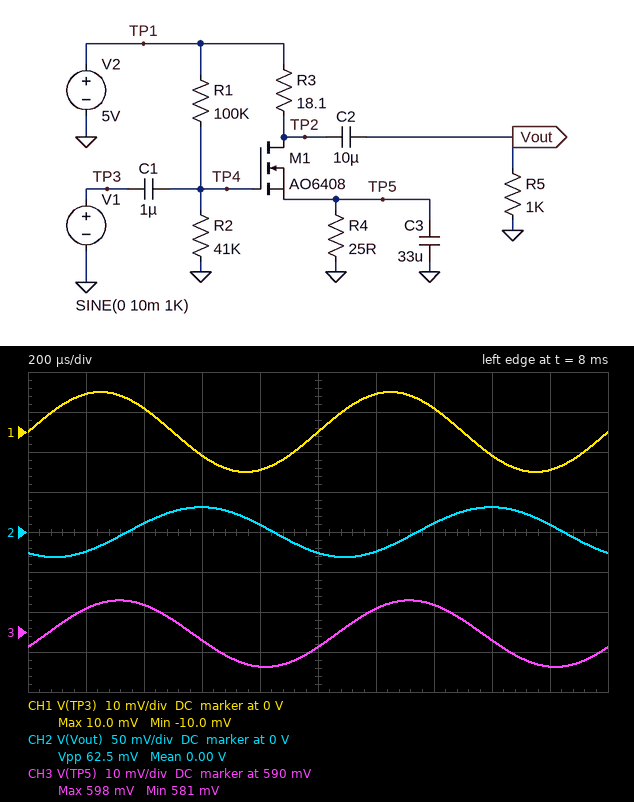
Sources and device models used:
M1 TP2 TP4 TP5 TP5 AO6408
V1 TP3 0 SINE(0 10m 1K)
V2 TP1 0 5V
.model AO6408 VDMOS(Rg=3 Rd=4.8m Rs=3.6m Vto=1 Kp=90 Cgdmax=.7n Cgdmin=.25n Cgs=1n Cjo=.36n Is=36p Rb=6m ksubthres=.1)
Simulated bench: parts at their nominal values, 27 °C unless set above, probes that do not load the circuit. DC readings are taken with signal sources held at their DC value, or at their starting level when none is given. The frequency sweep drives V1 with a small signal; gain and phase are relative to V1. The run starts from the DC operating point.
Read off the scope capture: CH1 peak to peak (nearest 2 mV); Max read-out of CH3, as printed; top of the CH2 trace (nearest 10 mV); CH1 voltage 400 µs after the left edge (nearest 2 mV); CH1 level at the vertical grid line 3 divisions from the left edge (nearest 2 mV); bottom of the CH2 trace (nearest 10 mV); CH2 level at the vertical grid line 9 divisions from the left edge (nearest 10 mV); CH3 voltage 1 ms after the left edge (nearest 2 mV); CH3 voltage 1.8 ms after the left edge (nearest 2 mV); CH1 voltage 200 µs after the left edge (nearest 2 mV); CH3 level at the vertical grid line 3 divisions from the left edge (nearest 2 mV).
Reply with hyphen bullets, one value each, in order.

- 20 mV
- 598 mV
- 30 mV
- 6 mV
- -6 mV
- -30 mV
- 10 mV
- 586 mV
- 582 mV
- 10 mV
- 588 mV
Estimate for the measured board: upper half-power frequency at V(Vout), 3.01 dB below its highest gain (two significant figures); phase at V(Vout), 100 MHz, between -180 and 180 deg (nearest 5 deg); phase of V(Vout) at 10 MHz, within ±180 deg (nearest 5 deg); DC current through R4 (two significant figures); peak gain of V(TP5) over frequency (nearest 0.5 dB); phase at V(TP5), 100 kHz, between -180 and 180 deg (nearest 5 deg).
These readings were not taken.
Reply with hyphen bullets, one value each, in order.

- 9.2 MHz
- 25 deg
- 125 deg
- 24 mA
- -1.0 dB
- -90 deg
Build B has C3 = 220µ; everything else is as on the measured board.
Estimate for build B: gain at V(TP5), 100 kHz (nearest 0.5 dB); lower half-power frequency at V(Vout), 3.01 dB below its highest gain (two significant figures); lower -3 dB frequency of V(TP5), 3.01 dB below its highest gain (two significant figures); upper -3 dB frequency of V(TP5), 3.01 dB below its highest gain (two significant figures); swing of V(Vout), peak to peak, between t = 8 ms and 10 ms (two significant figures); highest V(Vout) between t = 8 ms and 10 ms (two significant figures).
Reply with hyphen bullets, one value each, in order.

- -50.5 dB
- 330 Hz
- 5.3 Hz
- 340 Hz
- 140 mV
- 68 mV
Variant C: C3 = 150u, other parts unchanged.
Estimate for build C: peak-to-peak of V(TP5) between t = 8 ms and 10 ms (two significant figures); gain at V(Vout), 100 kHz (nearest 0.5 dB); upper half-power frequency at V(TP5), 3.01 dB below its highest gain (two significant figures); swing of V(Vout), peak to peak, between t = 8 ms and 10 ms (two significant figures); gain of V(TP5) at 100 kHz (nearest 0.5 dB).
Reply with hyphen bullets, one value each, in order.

- 8.0 mV
- 17.5 dB
- 500 Hz
- 130 mV
- -47.0 dB
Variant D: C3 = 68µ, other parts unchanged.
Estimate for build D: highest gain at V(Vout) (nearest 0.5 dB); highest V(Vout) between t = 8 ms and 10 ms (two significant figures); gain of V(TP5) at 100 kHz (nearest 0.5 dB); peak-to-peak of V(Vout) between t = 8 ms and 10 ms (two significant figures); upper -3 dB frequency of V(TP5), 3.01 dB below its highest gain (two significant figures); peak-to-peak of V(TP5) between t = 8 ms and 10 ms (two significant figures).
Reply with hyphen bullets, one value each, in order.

- 17.5 dB
- 50 mV
- -40.0 dB
- 100 mV
- 1.1 kHz
- 13 mV
